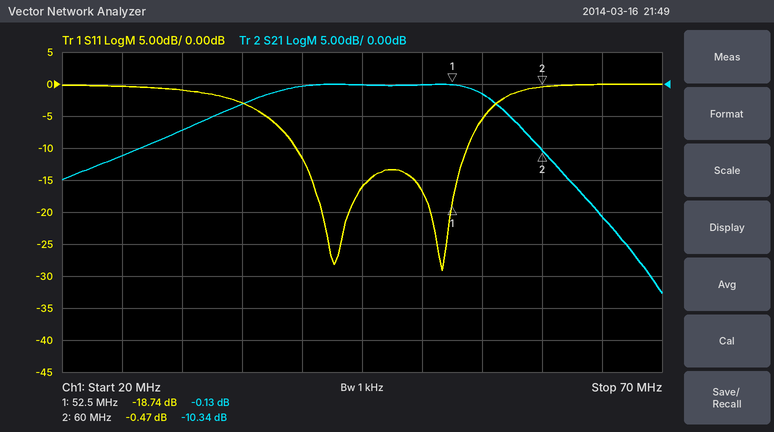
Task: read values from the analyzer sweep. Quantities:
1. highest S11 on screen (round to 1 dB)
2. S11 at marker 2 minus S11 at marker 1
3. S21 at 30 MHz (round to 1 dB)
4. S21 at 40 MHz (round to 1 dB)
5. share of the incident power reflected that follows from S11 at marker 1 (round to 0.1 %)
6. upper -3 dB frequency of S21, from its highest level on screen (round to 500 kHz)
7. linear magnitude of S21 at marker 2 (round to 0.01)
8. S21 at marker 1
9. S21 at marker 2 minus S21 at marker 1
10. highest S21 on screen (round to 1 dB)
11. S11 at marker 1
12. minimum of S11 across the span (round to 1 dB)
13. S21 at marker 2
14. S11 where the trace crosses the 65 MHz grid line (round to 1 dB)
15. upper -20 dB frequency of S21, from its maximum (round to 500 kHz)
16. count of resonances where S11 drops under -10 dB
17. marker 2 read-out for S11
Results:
0 dB
18.27 dB
-7 dB
0 dB
1.3 %
56.0 MHz
0.30
-0.13 dB
-10.21 dB
0 dB
-18.74 dB
-29 dB
-10.34 dB
0 dB
64.5 MHz
2
-0.47 dB
